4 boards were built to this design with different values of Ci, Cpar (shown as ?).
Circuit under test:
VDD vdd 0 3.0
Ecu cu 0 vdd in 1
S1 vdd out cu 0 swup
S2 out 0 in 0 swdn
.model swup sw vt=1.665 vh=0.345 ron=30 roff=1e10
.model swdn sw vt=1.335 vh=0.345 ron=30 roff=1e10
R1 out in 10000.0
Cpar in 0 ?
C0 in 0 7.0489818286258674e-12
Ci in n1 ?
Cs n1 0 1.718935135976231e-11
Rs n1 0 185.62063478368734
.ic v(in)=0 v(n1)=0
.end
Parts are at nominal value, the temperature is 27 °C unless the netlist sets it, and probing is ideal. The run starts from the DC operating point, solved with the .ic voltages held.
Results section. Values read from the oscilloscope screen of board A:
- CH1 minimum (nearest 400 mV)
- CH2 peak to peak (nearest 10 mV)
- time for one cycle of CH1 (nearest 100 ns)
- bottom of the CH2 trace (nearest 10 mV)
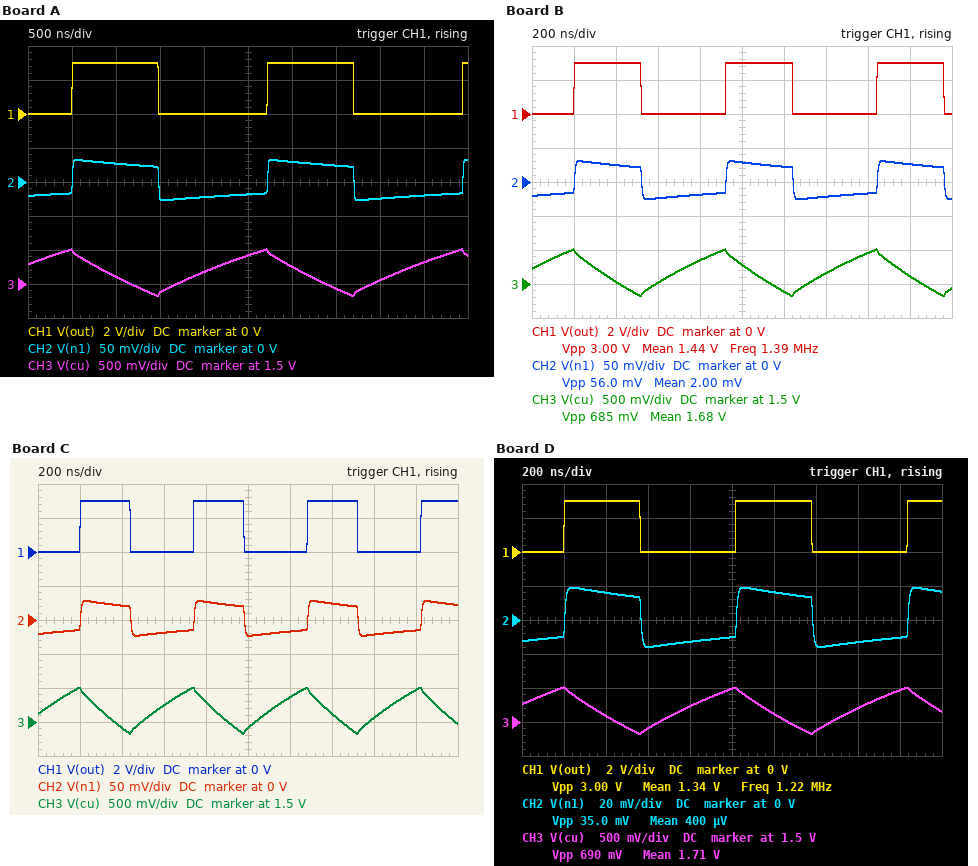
0 V
60 mV
2.2 µs
-30 mV
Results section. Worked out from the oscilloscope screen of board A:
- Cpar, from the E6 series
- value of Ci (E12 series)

15 pF
220 pF
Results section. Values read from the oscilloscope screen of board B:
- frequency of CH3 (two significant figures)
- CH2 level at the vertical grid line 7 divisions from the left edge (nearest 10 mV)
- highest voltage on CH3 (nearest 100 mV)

1.4 MHz
-20 mV
2.0 V
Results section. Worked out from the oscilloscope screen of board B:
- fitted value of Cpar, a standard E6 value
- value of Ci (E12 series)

3.3 pF
68 pF
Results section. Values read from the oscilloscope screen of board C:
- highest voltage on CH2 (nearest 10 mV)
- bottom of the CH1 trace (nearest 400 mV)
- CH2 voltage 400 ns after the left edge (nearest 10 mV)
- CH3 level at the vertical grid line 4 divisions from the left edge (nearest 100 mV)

30 mV
0 V
20 mV
1.8 V
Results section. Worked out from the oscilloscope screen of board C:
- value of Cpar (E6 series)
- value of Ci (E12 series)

4.7 pF
47 pF
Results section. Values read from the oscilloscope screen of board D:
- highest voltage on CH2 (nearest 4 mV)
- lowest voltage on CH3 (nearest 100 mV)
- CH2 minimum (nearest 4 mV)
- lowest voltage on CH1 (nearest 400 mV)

20 mV
1.3 V
-16 mV
0 V
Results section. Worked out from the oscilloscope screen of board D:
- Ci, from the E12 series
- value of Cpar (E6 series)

47 pF
33 pF
